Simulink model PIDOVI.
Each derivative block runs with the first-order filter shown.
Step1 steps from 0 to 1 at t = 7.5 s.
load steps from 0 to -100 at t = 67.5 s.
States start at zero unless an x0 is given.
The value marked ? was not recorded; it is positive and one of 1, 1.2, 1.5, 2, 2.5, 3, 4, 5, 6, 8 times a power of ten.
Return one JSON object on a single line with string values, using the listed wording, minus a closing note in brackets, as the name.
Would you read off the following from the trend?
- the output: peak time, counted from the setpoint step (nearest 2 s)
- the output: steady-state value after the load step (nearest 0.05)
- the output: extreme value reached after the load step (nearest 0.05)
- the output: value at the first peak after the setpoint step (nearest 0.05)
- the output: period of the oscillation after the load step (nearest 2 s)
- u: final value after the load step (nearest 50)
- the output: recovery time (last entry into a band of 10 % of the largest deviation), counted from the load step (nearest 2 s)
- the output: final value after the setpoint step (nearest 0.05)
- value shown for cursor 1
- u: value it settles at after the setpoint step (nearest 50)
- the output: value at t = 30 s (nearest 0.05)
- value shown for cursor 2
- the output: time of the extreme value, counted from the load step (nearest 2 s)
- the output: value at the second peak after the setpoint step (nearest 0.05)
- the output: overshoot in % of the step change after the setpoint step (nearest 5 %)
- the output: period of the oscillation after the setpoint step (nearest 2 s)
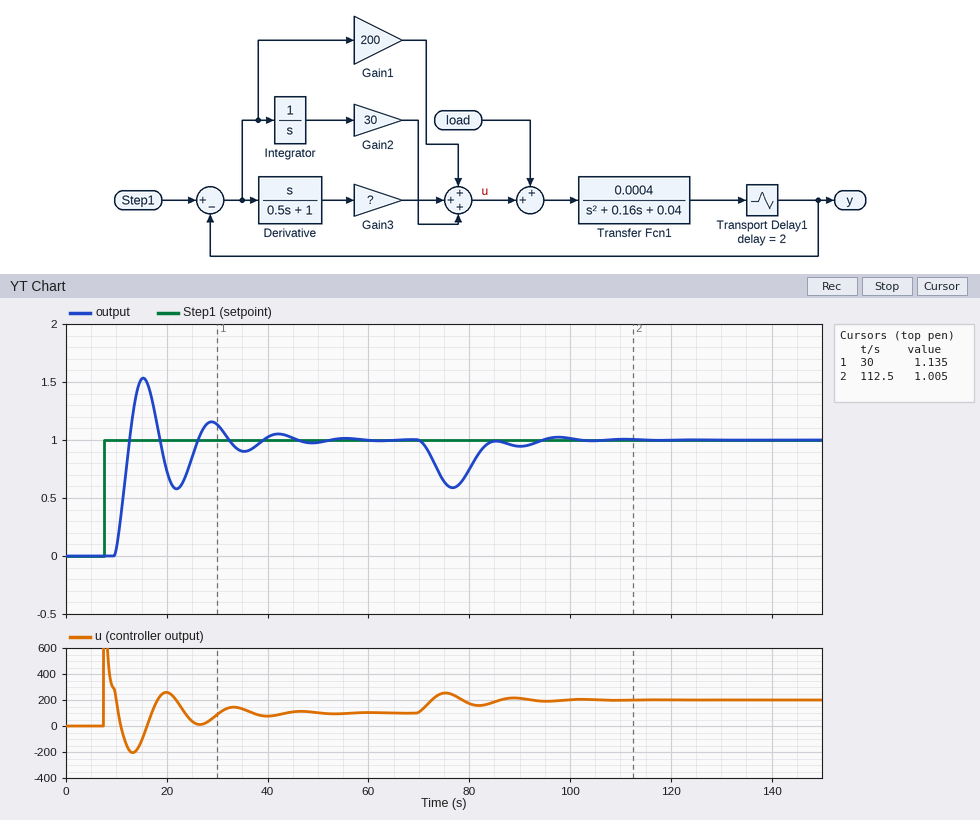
{"the output: peak time, counted from the setpoint step": "8 s", "the output: steady-state value after the load step": "1.00", "the output: extreme value reached after the load step": "0.60", "the output: value at the first peak after the setpoint step": "1.55", "the output: period of the oscillation after the load step": "14 s", "u: final value after the load step": "200", "the output: recovery time (last entry into a band of 10 % of the largest deviation), counted from the load step": "24 s", "the output: final value after the setpoint step": "1.00", "value shown for cursor 1": "1.135", "u: value it settles at after the setpoint step": "100", "the output: value at t = 30 s": "1.15", "value shown for cursor 2": "1.005", "the output: time of the extreme value, counted from the load step": "10 s", "the output: value at the second peak after the setpoint step": "1.15", "the output: overshoot in % of the step change after the setpoint step": "55 %", "the output: period of the oscillation after the setpoint step": "14 s"}
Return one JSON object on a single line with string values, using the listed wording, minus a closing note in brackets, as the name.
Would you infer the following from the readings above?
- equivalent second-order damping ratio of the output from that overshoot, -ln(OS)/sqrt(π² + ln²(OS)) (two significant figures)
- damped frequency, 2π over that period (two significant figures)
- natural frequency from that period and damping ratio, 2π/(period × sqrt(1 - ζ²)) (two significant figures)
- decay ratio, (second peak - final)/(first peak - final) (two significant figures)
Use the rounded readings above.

{"equivalent second-order damping ratio of the output from that overshoot, -ln(OS)/sqrt(π² + ln²(OS))": "0.19", "damped frequency, 2π over that period": "0.45 rad/s", "natural frequency from that period and damping ratio, 2π/(period × sqrt(1 - ζ²))": "0.46 rad/s", "decay ratio, (second peak - final)/(first peak - final)": "0.27"}
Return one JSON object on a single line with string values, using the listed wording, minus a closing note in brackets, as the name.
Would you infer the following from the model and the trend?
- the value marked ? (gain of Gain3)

{"the value marked ?": "800"}
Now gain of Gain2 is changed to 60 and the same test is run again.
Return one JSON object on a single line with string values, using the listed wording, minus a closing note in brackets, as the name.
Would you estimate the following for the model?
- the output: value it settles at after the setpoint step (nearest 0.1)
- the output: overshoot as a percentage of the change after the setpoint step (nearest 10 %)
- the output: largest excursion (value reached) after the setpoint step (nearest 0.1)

{"the output: value it settles at after the setpoint step": "1.0", "the output: overshoot as a percentage of the change after the setpoint step": "80 %", "the output: largest excursion (value reached) after the setpoint step": "1.8"}
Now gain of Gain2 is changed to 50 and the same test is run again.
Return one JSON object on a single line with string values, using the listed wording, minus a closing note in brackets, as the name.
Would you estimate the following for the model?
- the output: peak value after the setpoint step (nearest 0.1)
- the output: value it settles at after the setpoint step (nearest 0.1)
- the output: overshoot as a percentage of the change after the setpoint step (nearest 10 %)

{"the output: peak value after the setpoint step": "1.7", "the output: value it settles at after the setpoint step": "1.0", "the output: overshoot as a percentage of the change after the setpoint step": "70 %"}
